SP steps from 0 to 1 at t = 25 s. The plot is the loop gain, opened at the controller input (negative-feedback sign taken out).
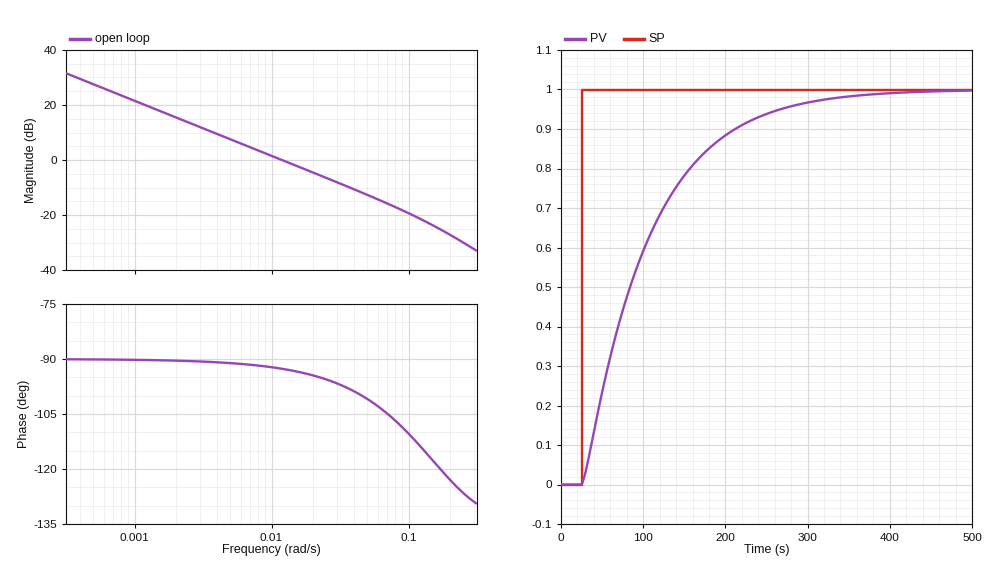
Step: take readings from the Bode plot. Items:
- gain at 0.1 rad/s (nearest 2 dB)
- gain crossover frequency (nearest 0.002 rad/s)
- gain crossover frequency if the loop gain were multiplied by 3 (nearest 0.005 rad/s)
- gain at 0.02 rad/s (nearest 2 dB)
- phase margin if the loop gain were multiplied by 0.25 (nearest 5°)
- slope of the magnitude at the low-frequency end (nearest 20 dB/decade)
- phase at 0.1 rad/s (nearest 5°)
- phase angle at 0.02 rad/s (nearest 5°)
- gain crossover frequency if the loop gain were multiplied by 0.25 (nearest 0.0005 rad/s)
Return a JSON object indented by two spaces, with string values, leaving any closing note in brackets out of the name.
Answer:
{
  "gain at 0.1 rad/s": "-20 dB",
  "gain crossover frequency": "0.012 rad/s",
  "gain crossover frequency if the loop gain were multiplied by 3": "0.035 rad/s",
  "gain at 0.02 rad/s": "-4 dB",
  "phase margin if the loop gain were multiplied by 0.25": "90°",
  "slope of the magnitude at the low-frequency end": "-20 dB/decade",
  "phase at 0.1 rad/s": "-110°",
  "phase angle at 0.02 rad/s": "-95°",
  "gain crossover frequency if the loop gain were multiplied by 0.25": "0.0030 rad/s"
}
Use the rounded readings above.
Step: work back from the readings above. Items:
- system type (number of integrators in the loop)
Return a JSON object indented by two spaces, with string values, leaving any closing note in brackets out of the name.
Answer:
{
  "system type": "1"
}
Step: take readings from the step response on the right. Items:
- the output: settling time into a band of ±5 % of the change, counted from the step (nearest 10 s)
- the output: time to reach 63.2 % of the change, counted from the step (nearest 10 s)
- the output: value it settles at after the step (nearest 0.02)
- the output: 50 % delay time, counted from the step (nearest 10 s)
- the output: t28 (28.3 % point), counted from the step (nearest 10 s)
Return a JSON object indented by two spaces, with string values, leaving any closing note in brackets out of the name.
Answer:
{
  "the output: settling time into a band of ±5 % of the change, counted from the step": "240 s",
  "the output: time to reach 63.2 % of the change, counted from the step": "80 s",
  "the output: value it settles at after the step": "1.00",
  "the output: 50 % delay time, counted from the step": "60 s",
  "the output: t28 (28.3 % point), counted from the step": "30 s"
}
